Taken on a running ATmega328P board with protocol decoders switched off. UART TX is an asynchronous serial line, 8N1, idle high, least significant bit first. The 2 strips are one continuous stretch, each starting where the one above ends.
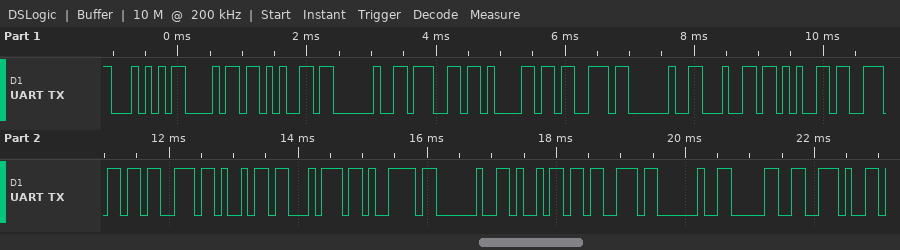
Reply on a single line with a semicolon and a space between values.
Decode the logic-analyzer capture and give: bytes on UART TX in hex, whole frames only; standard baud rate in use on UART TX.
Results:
54 68 65 20 67 61 73 20 64 65 6E 73 69 74 79 20 69 73 20 30 2E; 9600 baud
